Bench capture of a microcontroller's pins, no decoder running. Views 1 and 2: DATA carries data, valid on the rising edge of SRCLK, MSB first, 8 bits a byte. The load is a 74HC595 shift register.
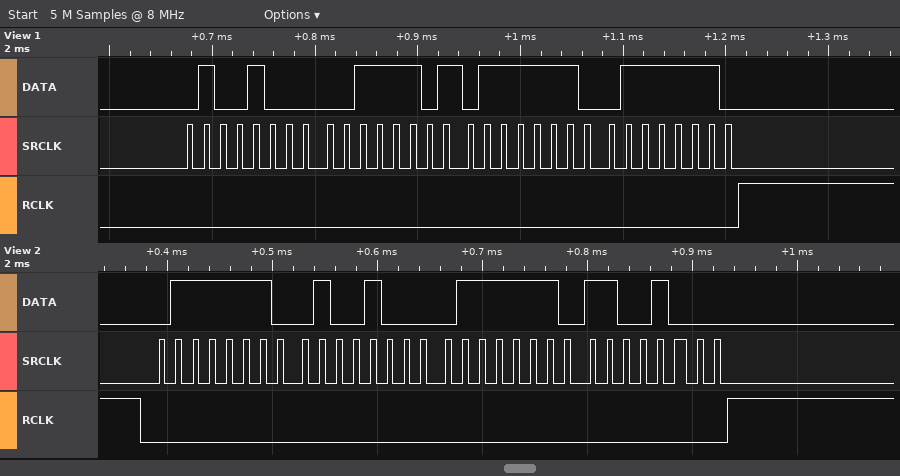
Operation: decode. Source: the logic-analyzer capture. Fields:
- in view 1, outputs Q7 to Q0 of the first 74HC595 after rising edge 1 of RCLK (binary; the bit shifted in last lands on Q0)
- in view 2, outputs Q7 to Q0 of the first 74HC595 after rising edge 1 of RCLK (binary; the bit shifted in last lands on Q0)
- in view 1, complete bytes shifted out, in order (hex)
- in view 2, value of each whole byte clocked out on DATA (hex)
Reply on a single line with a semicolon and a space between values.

01111110; 11001000; 48 3D 7E 7E; 0x7E 0x48 0x7E 0xC8
